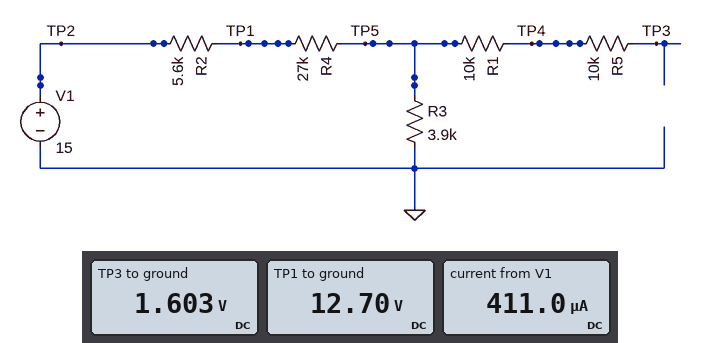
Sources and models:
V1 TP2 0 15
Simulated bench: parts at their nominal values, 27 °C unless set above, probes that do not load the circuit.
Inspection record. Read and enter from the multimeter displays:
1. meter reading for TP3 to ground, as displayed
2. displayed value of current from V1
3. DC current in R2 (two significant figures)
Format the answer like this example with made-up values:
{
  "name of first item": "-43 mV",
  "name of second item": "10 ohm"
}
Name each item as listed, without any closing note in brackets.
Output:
{
  "meter reading for TP3 to ground, as displayed": "1.603 V",
  "displayed value of current from V1": "411.0 µA",
  "DC current in R2": "410 µA"
}
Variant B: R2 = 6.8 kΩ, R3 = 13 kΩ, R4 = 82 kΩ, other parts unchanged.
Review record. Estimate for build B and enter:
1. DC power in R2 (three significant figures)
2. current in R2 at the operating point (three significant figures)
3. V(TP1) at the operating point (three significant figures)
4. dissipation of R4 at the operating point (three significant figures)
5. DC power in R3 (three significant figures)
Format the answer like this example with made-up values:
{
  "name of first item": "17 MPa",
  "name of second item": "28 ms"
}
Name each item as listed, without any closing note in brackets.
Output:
{
  "DC power in R2": "148 µW",
  "current in R2 at the operating point": "147 µA",
  "V(TP1) at the operating point": "14.0 V",
  "dissipation of R4 at the operating point": "1.78 mW",
  "DC power in R3": "282 µW"
}
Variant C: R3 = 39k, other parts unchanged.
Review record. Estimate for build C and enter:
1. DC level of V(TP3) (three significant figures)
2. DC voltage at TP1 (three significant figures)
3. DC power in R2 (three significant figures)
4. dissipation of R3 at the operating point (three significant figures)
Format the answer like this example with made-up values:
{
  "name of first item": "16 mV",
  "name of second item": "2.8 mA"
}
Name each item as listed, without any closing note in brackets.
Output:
{
  "DC level of V(TP3)": "8.17 V",
  "DC voltage at TP1": "13.8 V",
  "DC power in R2": "246 µW",
  "dissipation of R3 at the operating point": "1.71 mW"
}
